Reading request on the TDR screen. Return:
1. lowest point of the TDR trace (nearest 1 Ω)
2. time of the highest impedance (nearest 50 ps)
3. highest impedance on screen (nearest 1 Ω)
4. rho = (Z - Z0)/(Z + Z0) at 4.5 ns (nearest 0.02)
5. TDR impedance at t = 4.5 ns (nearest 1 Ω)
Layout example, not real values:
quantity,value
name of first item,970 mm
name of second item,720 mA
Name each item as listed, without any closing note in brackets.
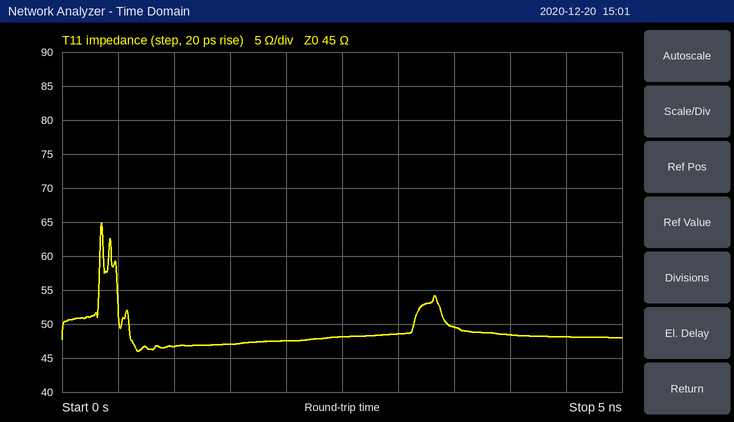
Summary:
quantity,value
lowest point of the TDR trace,46 Ω
time of the highest impedance,350 ps
highest impedance on screen,65 Ω
rho = (Z - Z0)/(Z + Z0) at 4.5 ns,+0.04
TDR impedance at t = 4.5 ns,48 Ω
